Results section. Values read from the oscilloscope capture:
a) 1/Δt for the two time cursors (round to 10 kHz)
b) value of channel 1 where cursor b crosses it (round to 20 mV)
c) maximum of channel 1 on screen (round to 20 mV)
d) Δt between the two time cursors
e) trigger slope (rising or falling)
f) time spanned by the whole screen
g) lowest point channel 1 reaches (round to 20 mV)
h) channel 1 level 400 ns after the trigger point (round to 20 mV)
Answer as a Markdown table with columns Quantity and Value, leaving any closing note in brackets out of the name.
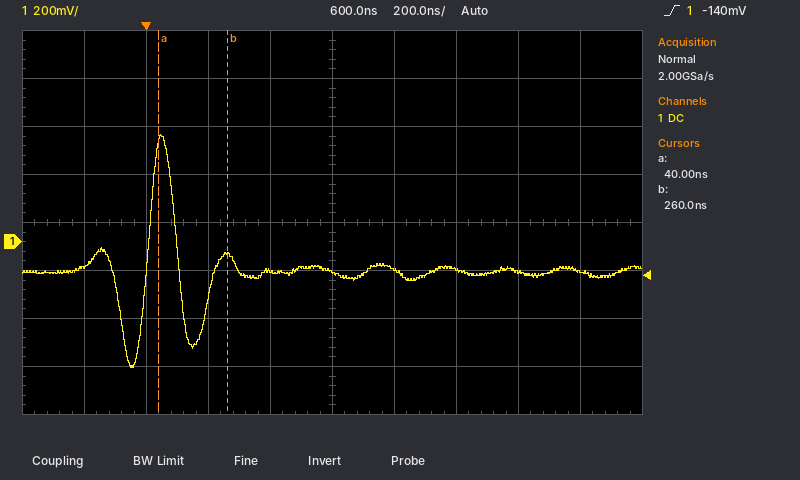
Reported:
| Quantity | Value |
|---|---|
| 1/Δt for the two time cursors | 4.55 MHz |
| value of channel 1 where cursor b crosses it | -60 mV |
| maximum of channel 1 on screen | 440 mV |
| Δt between the two time cursors | 220 ns |
| trigger slope | rising |
| time spanned by the whole screen | 2 µs |
| lowest point channel 1 reaches | -520 mV |
| channel 1 level 400 ns after the trigger point | -120 mV |
